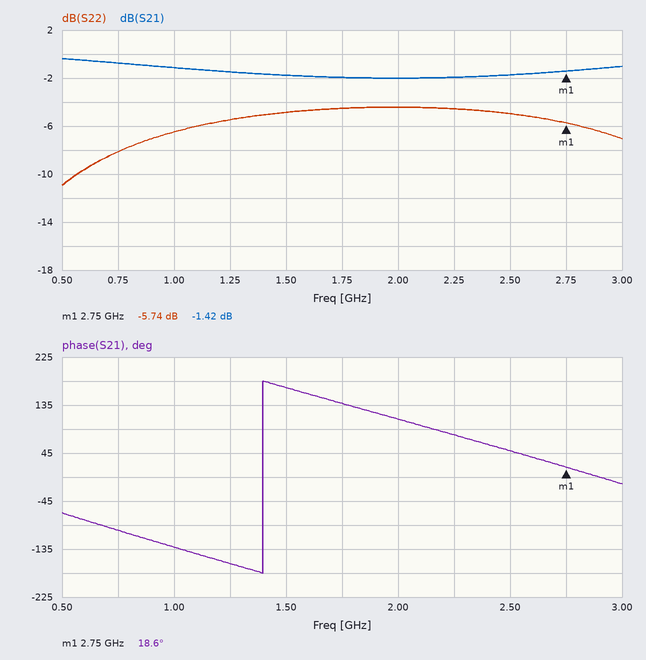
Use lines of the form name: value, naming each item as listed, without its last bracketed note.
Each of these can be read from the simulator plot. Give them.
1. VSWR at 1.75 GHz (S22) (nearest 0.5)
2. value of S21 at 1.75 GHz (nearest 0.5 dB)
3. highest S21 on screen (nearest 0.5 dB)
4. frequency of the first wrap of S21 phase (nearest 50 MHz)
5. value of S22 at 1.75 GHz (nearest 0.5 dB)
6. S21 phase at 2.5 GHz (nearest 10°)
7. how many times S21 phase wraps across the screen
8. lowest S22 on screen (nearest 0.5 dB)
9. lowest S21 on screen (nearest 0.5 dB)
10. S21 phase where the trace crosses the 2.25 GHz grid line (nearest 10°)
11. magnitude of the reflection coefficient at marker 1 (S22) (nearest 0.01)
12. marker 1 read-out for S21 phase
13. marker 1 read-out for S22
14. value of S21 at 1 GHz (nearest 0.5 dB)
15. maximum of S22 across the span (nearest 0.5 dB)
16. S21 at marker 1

VSWR at 1.75 GHz (S22): 4.0
value of S21 at 1.75 GHz: -2.0 dB
highest S21 on screen: -0.5 dB
frequency of the first wrap of S21 phase: 1.40 GHz
value of S22 at 1.75 GHz: -4.5 dB
S21 phase at 2.5 GHz: 50°
how many times S21 phase wraps across the screen: 1
lowest S22 on screen: -11.0 dB
lowest S21 on screen: -2.0 dB
S21 phase where the trace crosses the 2.25 GHz grid line: 80°
magnitude of the reflection coefficient at marker 1 (S22): 0.52
marker 1 read-out for S21 phase: 18.6°
marker 1 read-out for S22: -5.74 dB
value of S21 at 1 GHz: -1.0 dB
maximum of S22 across the span: -4.5 dB
S21 at marker 1: -1.42 dB
